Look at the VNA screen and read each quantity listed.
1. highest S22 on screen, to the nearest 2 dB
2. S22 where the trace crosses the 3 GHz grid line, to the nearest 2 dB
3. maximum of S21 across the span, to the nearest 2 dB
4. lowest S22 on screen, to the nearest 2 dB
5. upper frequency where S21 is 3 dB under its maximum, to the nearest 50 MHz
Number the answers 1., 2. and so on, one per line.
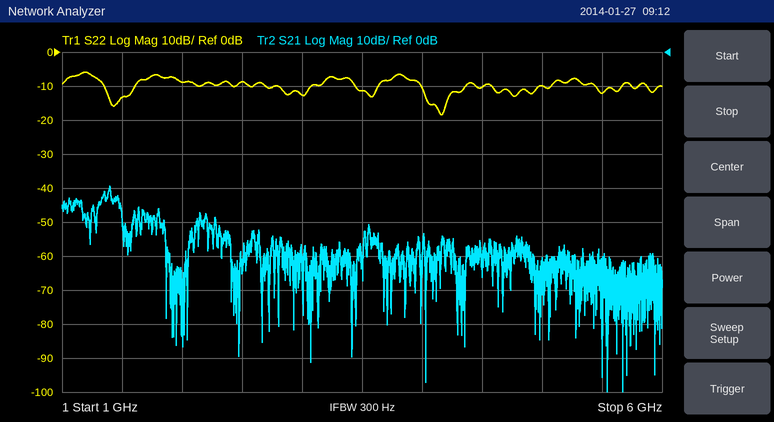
1. -6 dB
2. -12 dB
3. -40 dB
4. -18 dB
5. 1.40 GHz
